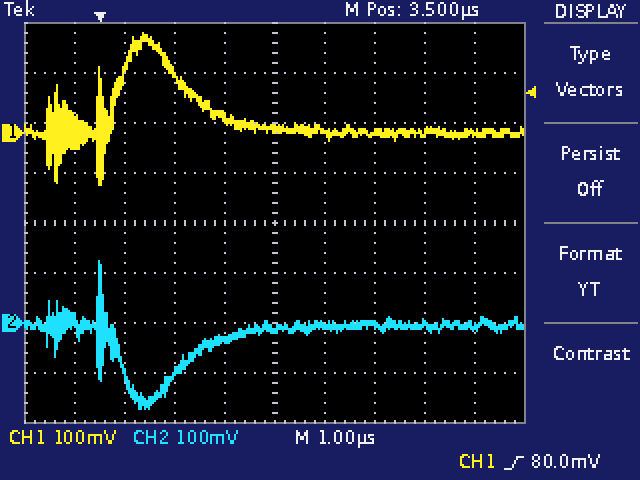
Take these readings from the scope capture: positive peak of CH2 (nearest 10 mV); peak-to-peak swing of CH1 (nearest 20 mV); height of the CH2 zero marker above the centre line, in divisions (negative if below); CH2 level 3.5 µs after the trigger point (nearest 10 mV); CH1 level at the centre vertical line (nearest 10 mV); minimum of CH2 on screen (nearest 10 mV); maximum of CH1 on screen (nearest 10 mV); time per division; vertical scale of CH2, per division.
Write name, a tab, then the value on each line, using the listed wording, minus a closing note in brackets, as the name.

positive peak of CH2	120 mV
peak-to-peak swing of CH1	300 mV
height of the CH2 zero marker above the centre line, in divisions	-2.0 div
CH2 level 3.5 µs after the trigger point	-10 mV
CH1 level at the centre vertical line	10 mV
minimum of CH2 on screen	-170 mV
maximum of CH1 on screen	200 mV
time per division	1 µs
vertical scale of CH2, per division	100 mV
